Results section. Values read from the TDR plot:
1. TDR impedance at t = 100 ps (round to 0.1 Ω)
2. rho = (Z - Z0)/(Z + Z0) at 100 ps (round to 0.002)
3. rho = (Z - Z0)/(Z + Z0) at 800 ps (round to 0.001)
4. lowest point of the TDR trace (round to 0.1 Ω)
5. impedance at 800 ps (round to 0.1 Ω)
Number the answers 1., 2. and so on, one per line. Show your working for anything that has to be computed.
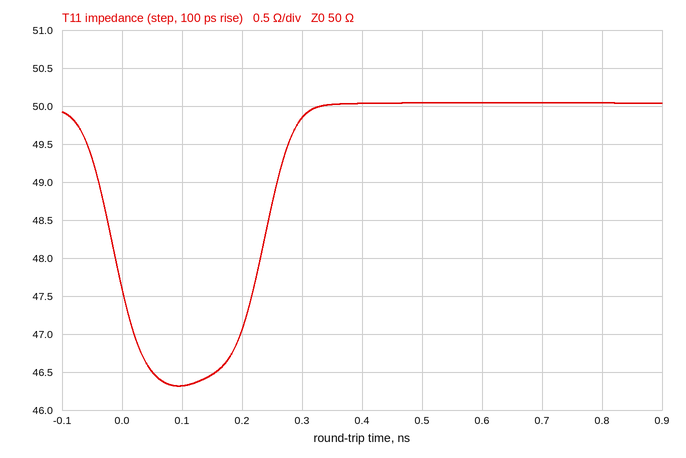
1. 46.3 Ω
2. (46.3 − 50)/(46.3 + 50) ≈ -0.038
3. (50 − 50)/(50 + 50) ≈ 0.000
4. 46.3 Ω
5. 50.0 Ω
